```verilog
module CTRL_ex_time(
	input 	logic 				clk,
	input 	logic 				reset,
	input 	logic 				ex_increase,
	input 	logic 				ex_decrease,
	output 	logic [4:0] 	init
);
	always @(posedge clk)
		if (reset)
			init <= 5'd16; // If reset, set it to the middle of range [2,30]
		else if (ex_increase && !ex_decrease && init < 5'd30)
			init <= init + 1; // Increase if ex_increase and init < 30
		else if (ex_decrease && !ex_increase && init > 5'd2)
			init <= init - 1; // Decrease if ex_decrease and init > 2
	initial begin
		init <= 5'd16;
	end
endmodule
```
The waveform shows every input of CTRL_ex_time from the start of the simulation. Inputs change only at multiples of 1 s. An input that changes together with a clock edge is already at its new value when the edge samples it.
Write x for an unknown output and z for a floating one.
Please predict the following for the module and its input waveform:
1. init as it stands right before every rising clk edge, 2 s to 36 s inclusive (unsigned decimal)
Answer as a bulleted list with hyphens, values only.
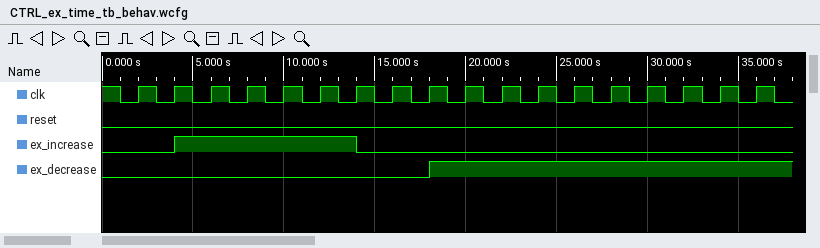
- 16, 16, 17, 18, 19, 20, 21, 21, 21, 20, 19, 18, 17, 16, 15, 14, 13, 12
